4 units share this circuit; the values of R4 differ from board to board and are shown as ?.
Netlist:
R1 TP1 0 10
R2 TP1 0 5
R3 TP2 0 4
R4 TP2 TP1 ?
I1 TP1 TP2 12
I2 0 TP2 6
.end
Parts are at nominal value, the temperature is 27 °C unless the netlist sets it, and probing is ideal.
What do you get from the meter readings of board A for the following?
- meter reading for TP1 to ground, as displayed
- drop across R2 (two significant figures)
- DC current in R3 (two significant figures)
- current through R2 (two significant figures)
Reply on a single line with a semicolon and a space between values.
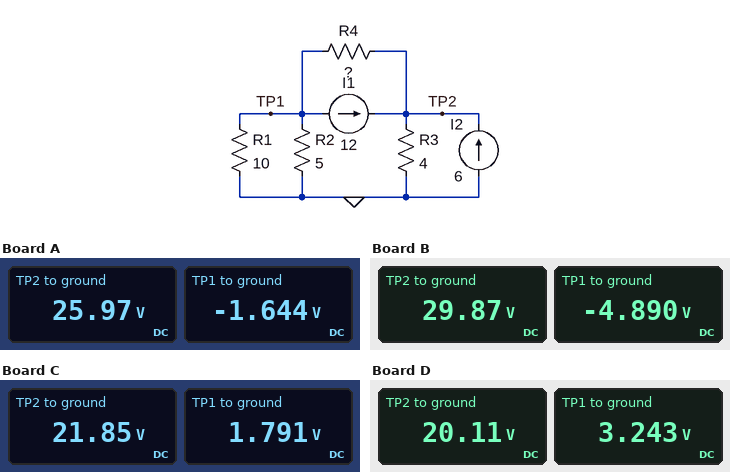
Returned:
-1.644 V; 1.6 V; 6.5 A; 330 mA
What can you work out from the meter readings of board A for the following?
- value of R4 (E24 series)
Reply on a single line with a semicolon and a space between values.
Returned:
2.4 Ω
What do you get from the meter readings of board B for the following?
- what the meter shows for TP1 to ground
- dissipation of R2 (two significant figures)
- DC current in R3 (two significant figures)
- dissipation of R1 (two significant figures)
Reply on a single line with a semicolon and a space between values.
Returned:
-4.890 V; 4.8 W; 7.5 A; 2.4 W
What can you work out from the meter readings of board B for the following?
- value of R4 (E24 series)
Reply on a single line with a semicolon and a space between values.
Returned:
3.3 Ω
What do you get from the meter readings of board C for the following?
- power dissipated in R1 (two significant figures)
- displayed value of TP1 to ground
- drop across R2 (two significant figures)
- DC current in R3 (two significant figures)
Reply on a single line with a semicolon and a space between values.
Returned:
320 mW; 1.791 V; 1.8 V; 5.5 A
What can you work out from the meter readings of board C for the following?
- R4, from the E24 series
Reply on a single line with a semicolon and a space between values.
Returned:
1.6 Ω
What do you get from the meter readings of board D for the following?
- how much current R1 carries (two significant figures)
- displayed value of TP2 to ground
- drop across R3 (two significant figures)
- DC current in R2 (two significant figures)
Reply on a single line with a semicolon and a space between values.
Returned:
320 mA; 20.11 V; 20 V; 650 mA
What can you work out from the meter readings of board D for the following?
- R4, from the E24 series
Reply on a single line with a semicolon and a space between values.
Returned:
1.3 Ω
